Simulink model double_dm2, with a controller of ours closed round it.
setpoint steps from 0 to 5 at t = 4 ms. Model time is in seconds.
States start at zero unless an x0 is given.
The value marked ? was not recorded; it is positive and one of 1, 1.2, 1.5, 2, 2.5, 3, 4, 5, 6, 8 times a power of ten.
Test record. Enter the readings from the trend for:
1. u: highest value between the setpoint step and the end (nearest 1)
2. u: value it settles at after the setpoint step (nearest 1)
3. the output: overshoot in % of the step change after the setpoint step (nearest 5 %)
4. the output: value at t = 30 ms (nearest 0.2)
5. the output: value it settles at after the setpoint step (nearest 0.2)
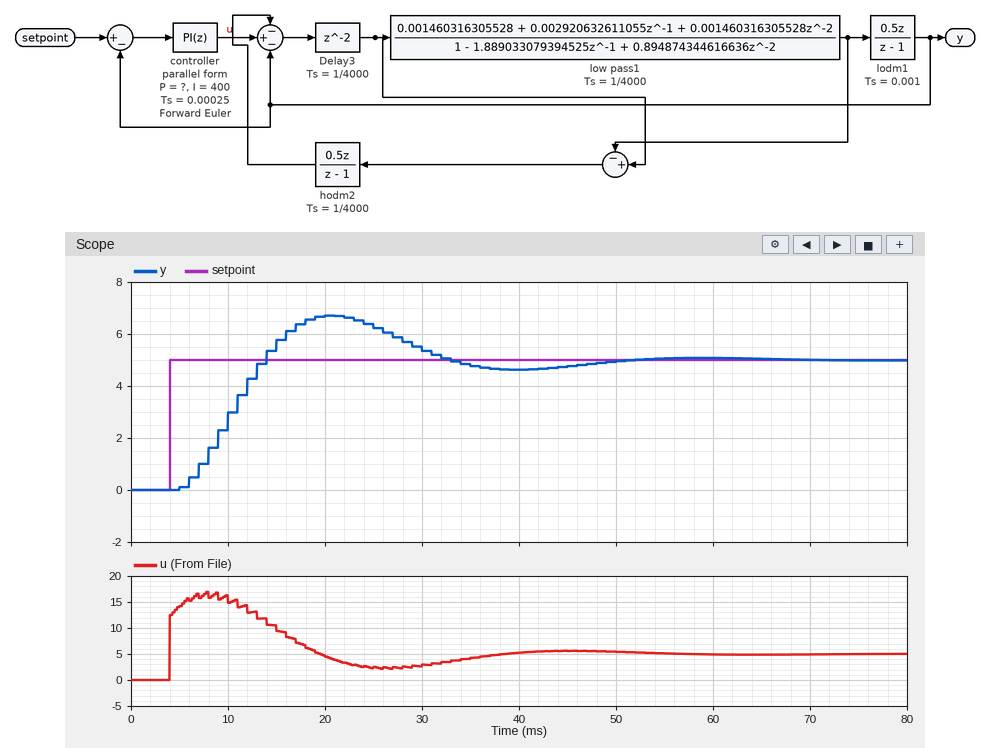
17
5
35 %
5.4
5.0
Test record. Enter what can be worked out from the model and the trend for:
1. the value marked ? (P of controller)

2.5
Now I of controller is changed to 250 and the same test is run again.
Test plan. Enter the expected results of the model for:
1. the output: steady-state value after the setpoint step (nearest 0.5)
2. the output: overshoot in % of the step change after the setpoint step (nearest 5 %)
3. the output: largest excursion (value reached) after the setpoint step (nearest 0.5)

5.0
15 %
6.0
